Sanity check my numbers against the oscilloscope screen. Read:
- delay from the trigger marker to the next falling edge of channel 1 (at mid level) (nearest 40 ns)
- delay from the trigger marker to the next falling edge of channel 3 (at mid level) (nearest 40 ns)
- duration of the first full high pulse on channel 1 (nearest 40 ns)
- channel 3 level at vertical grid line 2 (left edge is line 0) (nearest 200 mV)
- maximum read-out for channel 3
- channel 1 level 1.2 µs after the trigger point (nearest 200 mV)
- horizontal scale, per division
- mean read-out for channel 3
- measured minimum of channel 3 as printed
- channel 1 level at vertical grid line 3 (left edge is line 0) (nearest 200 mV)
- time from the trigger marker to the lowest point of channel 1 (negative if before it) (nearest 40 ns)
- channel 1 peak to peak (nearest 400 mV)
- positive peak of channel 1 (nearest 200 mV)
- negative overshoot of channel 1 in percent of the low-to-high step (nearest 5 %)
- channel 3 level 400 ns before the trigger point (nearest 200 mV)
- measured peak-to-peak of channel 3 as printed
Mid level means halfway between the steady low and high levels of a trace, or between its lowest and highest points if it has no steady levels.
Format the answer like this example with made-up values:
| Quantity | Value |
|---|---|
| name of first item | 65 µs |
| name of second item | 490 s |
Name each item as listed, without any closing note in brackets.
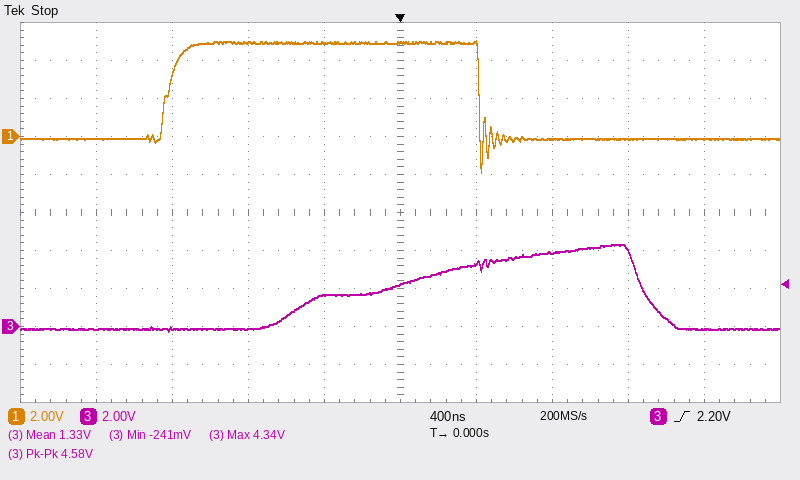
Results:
| Quantity | Value |
|---|---|
| delay from the trigger marker to the next falling edge of channel 1 (at mid level) | 400 ns |
| delay from the trigger marker to the next falling edge of channel 3 (at mid level) | 1.28 µs |
| duration of the first full high pulse on channel 1 | 1.64 µs |
| channel 3 level at vertical grid line 2 (left edge is line 0) | -200 mV |
| maximum read-out for channel 3 | 4.34 V |
| channel 1 level 1.2 µs after the trigger point | -200 mV |
| horizontal scale, per division | 400 ns |
| mean read-out for channel 3 | 1.33 V |
| measured minimum of channel 3 as printed | -241 mV |
| channel 1 level at vertical grid line 3 (left edge is line 0) | 5.0 V |
| time from the trigger marker to the lowest point of channel 1 (negative if before it) | +440 ns |
| channel 1 peak to peak | 6.8 V |
| positive peak of channel 1 | 5.0 V |
| negative overshoot of channel 1 in percent of the low-to-high step | 35 % |
| channel 3 level 400 ns before the trigger point | 1.6 V |
| measured peak-to-peak of channel 3 as printed | 4.58 V |
